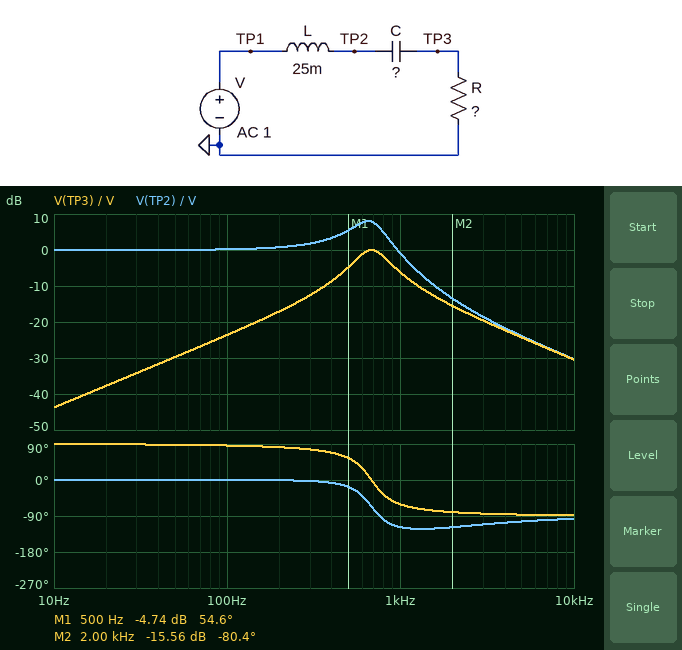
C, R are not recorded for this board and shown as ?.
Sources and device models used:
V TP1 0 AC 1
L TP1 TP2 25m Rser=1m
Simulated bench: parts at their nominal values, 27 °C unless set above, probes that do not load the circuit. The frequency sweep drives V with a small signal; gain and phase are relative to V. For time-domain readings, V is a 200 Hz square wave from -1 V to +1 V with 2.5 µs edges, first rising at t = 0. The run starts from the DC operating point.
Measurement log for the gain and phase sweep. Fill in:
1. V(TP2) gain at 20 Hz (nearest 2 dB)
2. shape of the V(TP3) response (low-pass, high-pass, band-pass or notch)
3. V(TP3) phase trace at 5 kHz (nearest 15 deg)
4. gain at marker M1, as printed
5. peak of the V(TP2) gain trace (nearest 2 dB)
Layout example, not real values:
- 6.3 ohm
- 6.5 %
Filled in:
- 0 dB
- band-pass
- -90 deg
- -4.74 dB
- 8 dB
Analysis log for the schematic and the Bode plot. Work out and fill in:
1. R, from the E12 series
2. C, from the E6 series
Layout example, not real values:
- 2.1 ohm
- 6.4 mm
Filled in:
- 47 Ω
- 2.2 µF
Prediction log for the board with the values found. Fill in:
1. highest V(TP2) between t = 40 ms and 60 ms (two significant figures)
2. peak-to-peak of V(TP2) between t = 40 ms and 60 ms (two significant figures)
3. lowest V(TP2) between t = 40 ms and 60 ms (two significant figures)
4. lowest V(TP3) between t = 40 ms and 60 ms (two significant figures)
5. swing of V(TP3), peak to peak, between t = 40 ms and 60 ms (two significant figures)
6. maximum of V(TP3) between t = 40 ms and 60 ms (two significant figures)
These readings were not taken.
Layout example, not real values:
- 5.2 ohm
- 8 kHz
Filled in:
- 2.2 V
- 4.3 V
- -2.2 V
- -700 mV
- 1.4 V
- 700 mV
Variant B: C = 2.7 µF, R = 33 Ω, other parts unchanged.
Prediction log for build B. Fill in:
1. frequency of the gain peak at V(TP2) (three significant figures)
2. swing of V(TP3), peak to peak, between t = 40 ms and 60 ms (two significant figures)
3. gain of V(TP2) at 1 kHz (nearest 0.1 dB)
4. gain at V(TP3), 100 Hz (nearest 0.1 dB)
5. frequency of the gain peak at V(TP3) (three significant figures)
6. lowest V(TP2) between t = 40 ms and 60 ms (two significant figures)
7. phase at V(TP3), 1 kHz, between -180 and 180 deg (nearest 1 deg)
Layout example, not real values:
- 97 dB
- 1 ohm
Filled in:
- 596 Hz
- 1.3 V
- -3.7 dB
- -24.8 dB
- 613 Hz
- -2.5 V
- -71 deg
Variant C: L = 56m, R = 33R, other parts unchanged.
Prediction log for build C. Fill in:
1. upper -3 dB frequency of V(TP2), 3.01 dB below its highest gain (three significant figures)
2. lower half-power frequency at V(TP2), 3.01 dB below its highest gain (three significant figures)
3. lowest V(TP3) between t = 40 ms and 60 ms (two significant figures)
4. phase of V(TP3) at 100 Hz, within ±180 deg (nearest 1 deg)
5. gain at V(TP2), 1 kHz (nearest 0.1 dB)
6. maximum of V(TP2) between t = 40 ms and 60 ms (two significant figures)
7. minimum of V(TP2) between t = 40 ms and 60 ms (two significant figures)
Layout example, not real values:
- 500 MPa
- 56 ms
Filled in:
- 494 Hz
- 399 Hz
- -250 mV
- 87 deg
- -11.0 dB
- 2.0 V
- -2.0 V
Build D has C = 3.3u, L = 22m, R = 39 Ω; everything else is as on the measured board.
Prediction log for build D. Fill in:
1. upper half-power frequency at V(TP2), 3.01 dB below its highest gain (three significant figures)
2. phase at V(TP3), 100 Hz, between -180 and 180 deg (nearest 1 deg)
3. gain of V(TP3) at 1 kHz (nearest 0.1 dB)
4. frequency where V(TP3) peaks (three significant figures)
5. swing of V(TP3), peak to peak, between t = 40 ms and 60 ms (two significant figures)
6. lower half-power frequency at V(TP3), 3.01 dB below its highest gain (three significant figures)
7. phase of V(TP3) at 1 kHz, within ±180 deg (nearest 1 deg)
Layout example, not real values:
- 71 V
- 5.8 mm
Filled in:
- 697 Hz
- 85 deg
- -8.0 dB
- 591 Hz
- 1.5 V
- 466 Hz
- -67 deg
